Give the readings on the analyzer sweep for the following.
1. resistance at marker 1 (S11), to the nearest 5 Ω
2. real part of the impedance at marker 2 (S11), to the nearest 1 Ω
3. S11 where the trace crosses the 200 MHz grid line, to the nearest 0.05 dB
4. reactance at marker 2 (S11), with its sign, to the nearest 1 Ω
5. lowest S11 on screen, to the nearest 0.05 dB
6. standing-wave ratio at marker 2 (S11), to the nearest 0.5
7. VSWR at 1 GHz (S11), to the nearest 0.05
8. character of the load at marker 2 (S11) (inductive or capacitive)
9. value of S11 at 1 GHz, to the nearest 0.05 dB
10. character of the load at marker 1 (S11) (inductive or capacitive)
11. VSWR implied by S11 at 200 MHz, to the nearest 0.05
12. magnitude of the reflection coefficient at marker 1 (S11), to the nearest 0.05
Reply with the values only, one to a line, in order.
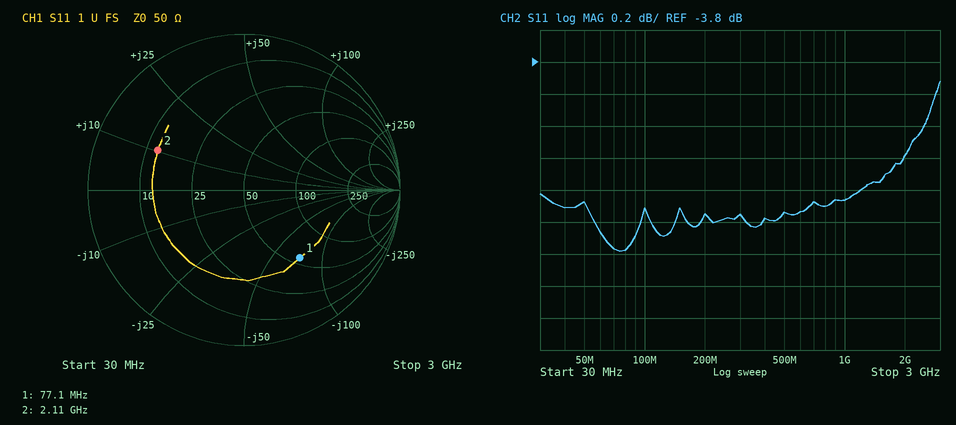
55 Ω
13 Ω
-4.75 dB
+10 Ω
-5.00 dB
4.0
3.80
inductive
-4.65 dB
capacitive
3.75
0.55
